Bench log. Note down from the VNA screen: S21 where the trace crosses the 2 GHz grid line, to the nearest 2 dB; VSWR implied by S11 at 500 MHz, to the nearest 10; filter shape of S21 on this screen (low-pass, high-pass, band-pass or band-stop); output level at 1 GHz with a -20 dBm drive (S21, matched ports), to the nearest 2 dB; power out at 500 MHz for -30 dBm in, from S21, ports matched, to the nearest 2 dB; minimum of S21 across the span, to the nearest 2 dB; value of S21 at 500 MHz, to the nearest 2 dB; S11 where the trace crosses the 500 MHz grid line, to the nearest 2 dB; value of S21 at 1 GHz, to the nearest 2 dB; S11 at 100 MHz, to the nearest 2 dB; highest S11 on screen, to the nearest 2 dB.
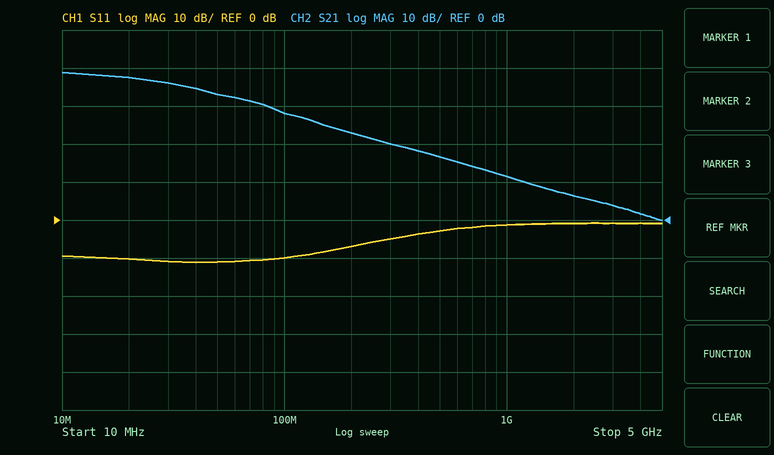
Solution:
6 dB
10
low-pass
-8 dBm
-14 dBm
0 dB
16 dB
-2 dB
12 dB
-10 dB
0 dB
